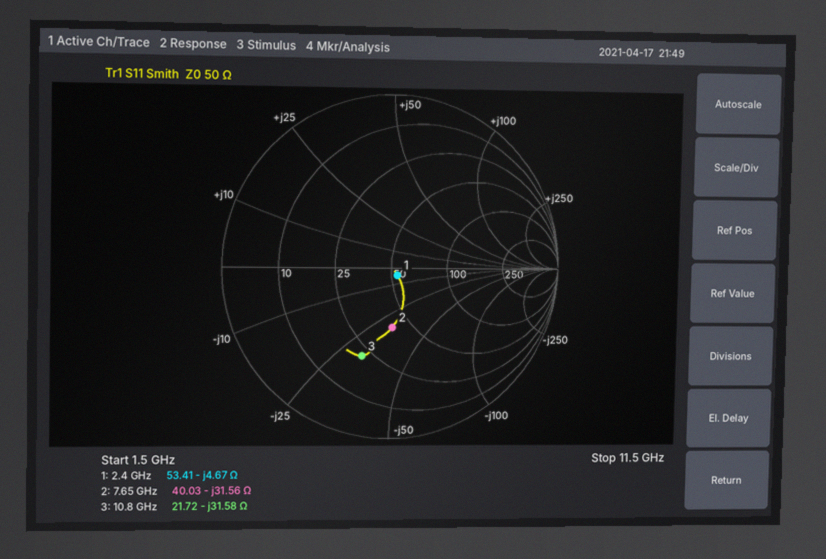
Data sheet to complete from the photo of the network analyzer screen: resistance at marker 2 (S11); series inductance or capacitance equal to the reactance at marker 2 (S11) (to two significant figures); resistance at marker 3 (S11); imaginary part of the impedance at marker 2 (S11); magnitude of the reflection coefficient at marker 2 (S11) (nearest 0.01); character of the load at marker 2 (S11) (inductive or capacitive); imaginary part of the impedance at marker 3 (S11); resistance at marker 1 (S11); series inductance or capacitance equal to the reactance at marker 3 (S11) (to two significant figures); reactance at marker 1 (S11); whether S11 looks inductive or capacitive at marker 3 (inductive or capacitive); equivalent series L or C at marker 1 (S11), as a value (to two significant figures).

40.03 Ω
660 fF
21.72 Ω
-31.56 Ω
0.35
capacitive
-31.58 Ω
53.41 Ω
470 fF
-4.67 Ω
capacitive
14 pF
